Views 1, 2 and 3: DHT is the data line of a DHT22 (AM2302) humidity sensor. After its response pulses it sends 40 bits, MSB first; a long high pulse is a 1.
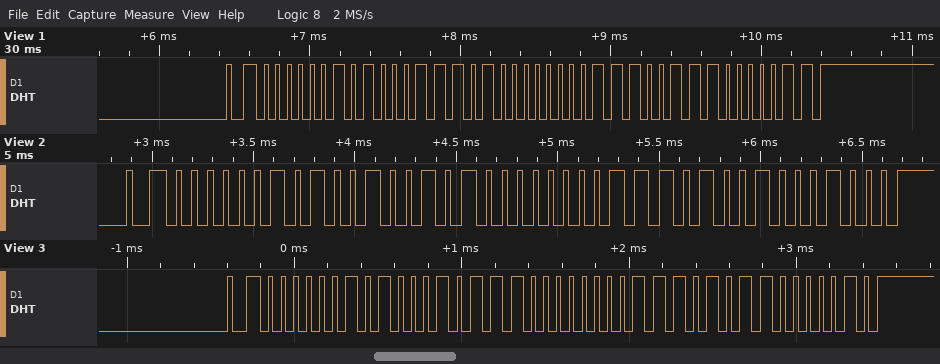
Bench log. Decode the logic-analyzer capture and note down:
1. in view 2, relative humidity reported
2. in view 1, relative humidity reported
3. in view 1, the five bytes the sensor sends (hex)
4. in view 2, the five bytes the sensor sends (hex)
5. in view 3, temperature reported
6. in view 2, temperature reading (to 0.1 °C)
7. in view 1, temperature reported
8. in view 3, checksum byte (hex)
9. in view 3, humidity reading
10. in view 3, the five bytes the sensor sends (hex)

65.8 %
65.4 %
02 8E 80 73 83
02 92 80 74 88
-11.7 °C
-11.6 °C
-11.5 °C
0x82
65.1 %
02 8B 80 75 82
